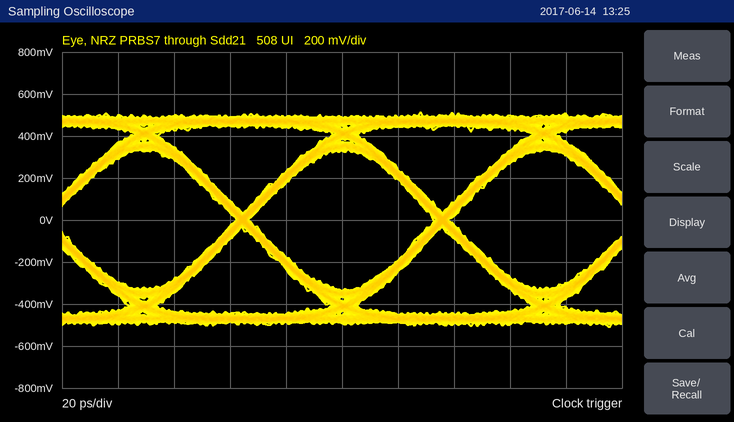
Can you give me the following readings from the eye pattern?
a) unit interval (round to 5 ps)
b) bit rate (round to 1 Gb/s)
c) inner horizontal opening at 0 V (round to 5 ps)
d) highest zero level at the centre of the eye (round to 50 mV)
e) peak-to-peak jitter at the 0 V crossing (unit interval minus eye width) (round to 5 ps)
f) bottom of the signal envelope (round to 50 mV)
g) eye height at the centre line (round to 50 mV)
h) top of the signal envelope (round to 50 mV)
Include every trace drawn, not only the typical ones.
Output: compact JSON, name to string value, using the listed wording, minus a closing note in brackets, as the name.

{"unit interval": "70 ps", "bit rate": "14 Gb/s", "inner horizontal opening at 0 V": "65 ps", "highest zero level at the centre of the eye": "-350 mV", "peak-to-peak jitter at the 0 V crossing (unit interval minus eye width)": "5 ps", "bottom of the signal envelope": "-500 mV", "eye height at the centre line": "650 mV", "top of the signal envelope": "500 mV"}
